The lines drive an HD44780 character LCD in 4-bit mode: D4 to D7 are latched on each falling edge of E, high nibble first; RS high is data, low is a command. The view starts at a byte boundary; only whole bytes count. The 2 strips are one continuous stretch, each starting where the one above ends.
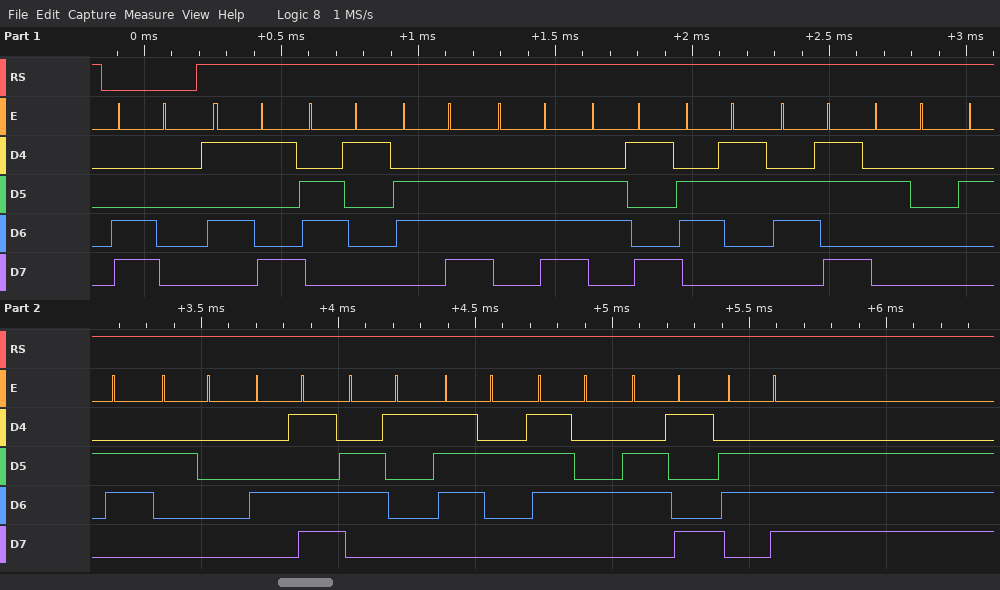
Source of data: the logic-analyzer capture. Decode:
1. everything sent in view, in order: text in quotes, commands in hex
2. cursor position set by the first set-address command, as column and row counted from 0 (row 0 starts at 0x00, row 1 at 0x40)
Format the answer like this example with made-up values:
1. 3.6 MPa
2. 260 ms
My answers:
1. 0xC0 "Yannick & Martin"
2. column 0, row 1
